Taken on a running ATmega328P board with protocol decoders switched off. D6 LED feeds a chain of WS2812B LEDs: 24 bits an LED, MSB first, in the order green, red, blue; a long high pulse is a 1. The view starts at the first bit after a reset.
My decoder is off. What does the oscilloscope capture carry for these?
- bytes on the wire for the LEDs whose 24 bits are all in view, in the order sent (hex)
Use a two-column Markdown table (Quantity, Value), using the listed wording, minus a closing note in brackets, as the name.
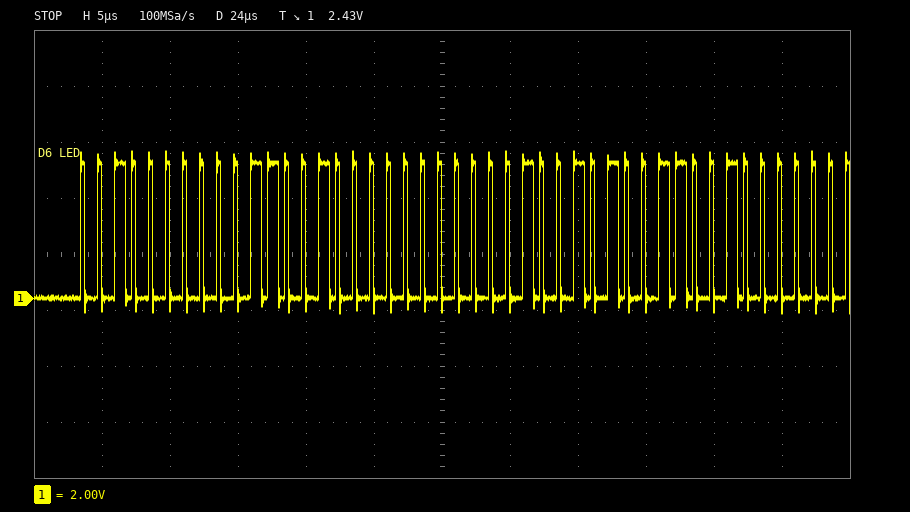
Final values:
| Quantity | Value |
|---|---|
| bytes on the wire for the LEDs whose 24 bits are all in view, in the order sent | 20 32 00 |
